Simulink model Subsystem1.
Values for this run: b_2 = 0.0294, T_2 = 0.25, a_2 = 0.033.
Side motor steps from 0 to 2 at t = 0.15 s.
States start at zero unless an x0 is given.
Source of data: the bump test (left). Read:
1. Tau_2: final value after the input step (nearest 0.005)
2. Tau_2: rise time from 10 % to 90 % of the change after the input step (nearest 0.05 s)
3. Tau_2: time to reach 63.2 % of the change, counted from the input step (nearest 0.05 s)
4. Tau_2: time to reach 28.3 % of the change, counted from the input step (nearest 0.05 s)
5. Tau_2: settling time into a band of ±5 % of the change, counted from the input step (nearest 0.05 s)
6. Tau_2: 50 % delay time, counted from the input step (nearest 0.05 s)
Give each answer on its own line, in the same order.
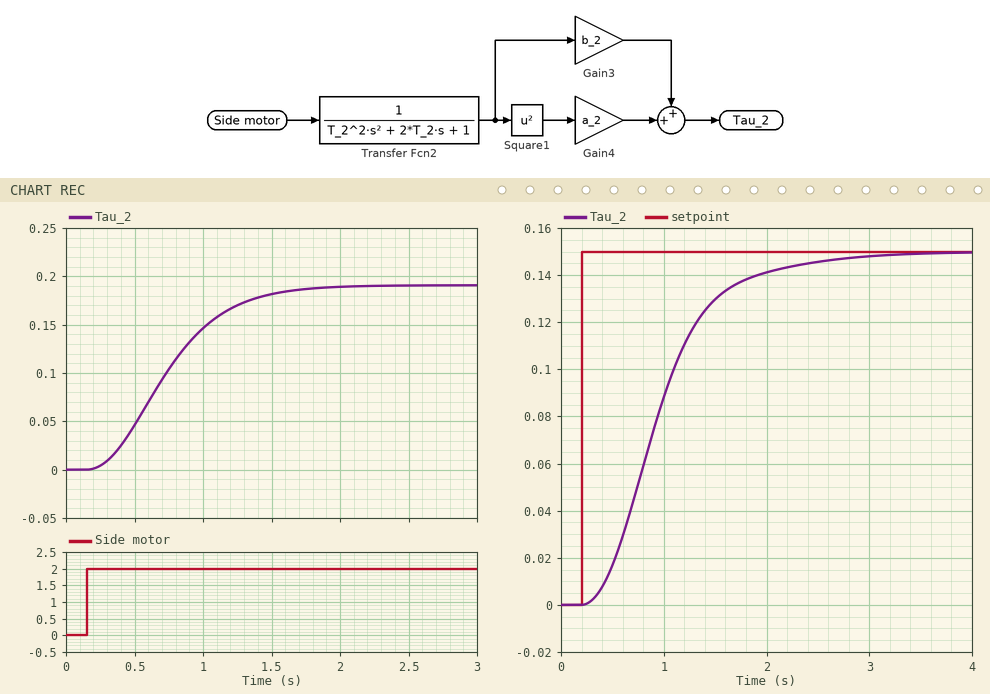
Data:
0.190
0.90 s
0.70 s
0.40 s
1.35 s
0.55 s
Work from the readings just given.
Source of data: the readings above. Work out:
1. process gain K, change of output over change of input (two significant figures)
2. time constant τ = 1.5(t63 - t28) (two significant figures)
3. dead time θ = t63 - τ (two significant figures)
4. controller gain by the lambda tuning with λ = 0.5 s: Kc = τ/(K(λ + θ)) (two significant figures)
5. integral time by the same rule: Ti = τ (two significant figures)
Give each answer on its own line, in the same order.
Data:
0.095
0.45 s
0.25 s
6.3
0.45 s
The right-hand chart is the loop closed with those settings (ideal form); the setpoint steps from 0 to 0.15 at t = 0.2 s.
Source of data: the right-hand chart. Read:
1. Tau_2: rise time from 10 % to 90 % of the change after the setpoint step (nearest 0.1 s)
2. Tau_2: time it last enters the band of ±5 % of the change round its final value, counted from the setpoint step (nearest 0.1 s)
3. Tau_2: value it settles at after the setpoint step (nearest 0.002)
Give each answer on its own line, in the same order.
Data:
1.2 s
1.9 s
0.150
